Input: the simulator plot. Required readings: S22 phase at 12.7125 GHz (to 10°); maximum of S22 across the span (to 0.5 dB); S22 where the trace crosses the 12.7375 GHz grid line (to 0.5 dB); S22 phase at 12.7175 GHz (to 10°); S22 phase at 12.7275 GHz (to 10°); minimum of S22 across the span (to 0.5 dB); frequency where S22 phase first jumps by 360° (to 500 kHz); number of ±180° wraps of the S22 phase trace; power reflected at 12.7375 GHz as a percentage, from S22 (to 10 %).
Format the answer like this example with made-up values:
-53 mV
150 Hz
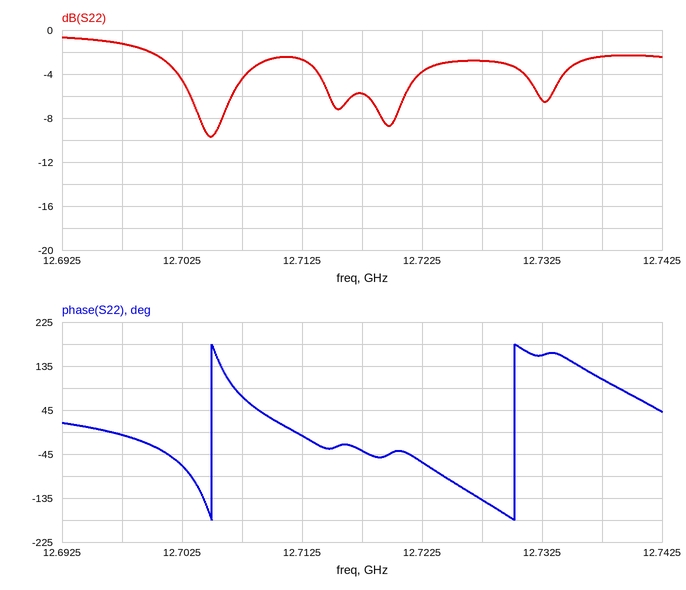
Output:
-10°
-0.5 dB
-2.5 dB
-40°
-140°
-9.5 dB
12.7050 GHz
2
60 %
